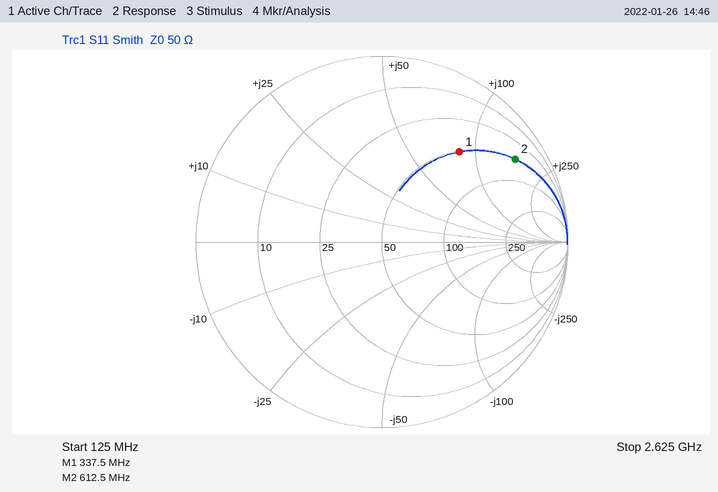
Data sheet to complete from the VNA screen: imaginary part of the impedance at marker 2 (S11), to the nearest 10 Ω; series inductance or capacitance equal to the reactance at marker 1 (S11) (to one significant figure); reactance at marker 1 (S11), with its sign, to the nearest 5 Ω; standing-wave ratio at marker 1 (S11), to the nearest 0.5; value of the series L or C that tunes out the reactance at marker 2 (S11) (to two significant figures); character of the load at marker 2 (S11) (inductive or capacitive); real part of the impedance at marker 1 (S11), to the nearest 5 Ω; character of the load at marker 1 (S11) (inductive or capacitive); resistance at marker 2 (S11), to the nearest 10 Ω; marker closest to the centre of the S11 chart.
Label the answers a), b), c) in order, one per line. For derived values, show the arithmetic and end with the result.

a) +160 Ω
b) L = 85 Ω/(2π × 337.5 MHz) ≈ 40 nH
c) +85 Ω
d) 4.5
e) C = 1/(2π × 612.5 MHz × 160 Ω) ≈ 1.6 pF
f) inductive
g) 50 Ω
h) inductive
i) 50 Ω
j) marker 1
